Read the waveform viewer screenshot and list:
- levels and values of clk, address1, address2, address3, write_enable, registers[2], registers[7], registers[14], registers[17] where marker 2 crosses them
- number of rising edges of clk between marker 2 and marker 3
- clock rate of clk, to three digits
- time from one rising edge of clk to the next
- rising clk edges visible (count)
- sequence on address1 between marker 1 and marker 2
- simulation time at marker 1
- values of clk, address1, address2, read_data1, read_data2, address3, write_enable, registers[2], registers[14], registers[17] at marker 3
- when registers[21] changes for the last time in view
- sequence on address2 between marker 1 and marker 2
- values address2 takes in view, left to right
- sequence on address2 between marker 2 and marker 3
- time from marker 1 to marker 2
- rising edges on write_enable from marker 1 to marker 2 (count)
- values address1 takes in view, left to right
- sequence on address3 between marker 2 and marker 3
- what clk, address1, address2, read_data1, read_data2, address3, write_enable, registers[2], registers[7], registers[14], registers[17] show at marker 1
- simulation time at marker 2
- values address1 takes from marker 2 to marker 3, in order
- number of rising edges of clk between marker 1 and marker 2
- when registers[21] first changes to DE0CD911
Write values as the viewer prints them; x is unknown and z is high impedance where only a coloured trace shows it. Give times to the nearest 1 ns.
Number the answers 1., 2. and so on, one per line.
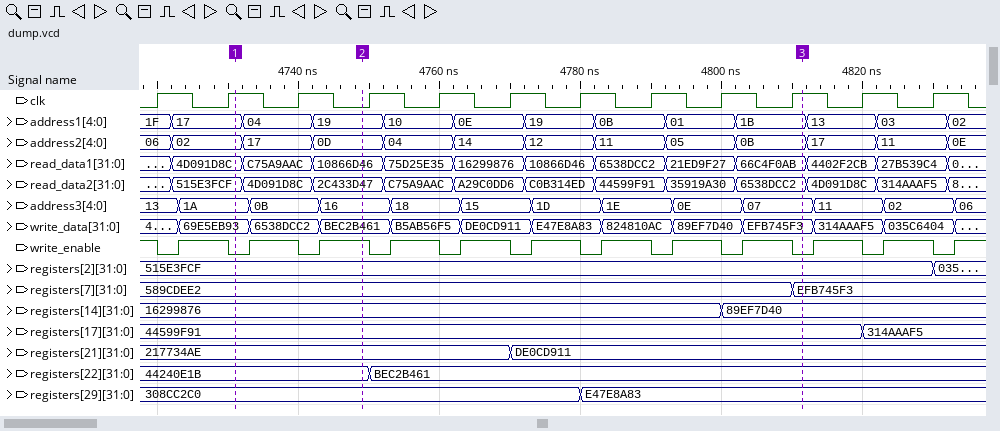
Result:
1. clk=0, address1=19, address2=0D, address3=16, write_enable=1, registers[2]=515E3FCF, registers[7]=589CDEE2, registers[14]=16299876, registers[17]=44599F91
2. 7
3. 100 MHz
4. 10 ns
5. 12
6. 17, 04, 19
7. 4731 ns
8. clk=1, address1=1B, address2=0B, read_data1=66C4F0AB, read_data2=6538DCC2, address3=07, write_enable=0, registers[2]=515E3FCF, registers[14]=89EF7D40, registers[17]=44599F91
9. 4770 ns
10. 02, 17, 0D
11. 06, 02, 17, 0D, 04, 14, 12, 11, 05, 0B, 17, 11, 0E
12. 0D, 04, 14, 12, 11, 05, 0B
13. 18 ns
14. 2
15. 1F, 17, 04, 19, 10, 0E, 19, 0B, 01, 1B, 13, 03, 02
16. 16, 18, 15, 1D, 1E, 0E, 07
17. clk=1, address1=17, address2=02, read_data1=4D091D8C, read_data2=515E3FCF, address3=1A, write_enable=0, registers[2]=515E3FCF, registers[7]=589CDEE2, registers[14]=16299876, registers[17]=44599F91
18. 4749 ns
19. 19, 10, 0E, 19, 0B, 01, 1B
20. 1
21. 4770 ns
